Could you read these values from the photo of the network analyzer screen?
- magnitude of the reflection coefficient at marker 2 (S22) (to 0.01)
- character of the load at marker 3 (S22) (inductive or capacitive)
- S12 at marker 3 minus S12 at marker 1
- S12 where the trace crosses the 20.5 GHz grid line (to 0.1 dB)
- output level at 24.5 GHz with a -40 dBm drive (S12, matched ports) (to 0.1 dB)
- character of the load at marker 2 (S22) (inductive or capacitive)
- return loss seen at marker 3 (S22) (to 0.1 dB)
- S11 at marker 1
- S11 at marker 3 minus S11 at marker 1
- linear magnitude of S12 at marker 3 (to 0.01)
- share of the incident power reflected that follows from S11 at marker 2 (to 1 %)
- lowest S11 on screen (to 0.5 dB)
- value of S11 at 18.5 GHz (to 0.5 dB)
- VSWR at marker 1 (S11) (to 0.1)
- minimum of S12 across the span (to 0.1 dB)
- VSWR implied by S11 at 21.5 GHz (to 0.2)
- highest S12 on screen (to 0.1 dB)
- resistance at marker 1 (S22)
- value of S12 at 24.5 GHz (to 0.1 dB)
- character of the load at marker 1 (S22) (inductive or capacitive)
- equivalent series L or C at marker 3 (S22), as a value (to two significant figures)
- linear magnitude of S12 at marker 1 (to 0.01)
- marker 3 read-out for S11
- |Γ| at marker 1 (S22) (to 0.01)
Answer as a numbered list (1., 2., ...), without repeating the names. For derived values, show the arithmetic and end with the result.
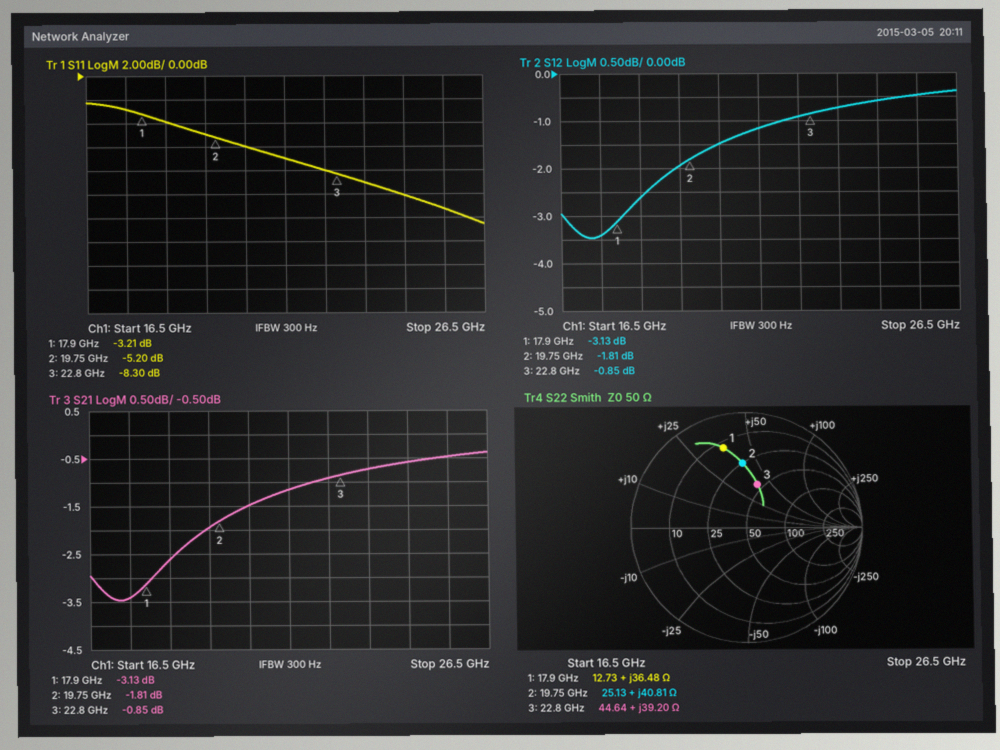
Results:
1. 0.56
2. inductive
3. -0.85 − (-3.13) = 2.28 dB
4. -1.5 dB
5. -40 dBm + (-0.6 dB) = -40.6 dBm
6. inductive
7. 8.3 dB
8. -3.21 dB
9. -8.3 − (-3.21) = -5.09 dB
10. 10^(-0.85/20) ≈ 0.91
11. 10^(-5.2/10) ≈ 30 %
12. -12.5 dB
13. -4.0 dB
14. (1 + 0.6910)/(1 − 0.6910) ≈ 5.5
15. -3.5 dB
16. |Γ| = 10^(-7/20) = 0.4467; VSWR = (1 + 0.4467)/(1 − 0.4467) ≈ 2.6
17. -0.4 dB
18. 12.73 Ω
19. -0.6 dB
20. inductive
21. L = 39.2 Ω/(2π × 22.8 GHz) ≈ 274 pH, so 270 pH to two significant figures
22. 10^(-3.13/20) ≈ 0.70
23. -8.30 dB
24. 0.72
